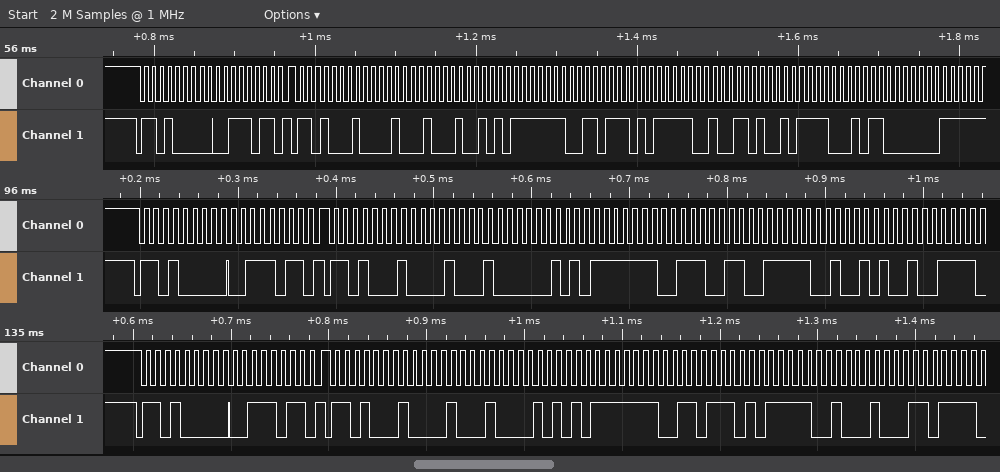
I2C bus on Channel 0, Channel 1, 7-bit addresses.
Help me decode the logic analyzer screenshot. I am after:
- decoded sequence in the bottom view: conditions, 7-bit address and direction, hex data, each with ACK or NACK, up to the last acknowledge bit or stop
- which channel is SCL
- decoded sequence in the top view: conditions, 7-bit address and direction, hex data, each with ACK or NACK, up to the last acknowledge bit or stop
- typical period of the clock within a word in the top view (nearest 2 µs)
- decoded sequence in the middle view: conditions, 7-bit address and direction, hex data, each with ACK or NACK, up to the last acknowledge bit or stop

start, address 68 write ACK, 3B ACK, repeated start, address 68 read ACK, 11 ACK, 15 ACK, FE ACK, DD ACK, F9 ACK, 23 ACK
Channel 0
start, address 68 write ACK, 3B ACK, repeated start, address 68 read ACK, 11 ACK, 25 ACK, FE ACK, DD ACK, F9 ACK, 69 ACK, F1 ACK, C0 ACK
10 µs
start, address 68 write ACK, 3B ACK, repeated start, address 68 read ACK, 11 ACK, 05 ACK, FE ACK, E6 ACK, F9 ACK, 52 ACK
